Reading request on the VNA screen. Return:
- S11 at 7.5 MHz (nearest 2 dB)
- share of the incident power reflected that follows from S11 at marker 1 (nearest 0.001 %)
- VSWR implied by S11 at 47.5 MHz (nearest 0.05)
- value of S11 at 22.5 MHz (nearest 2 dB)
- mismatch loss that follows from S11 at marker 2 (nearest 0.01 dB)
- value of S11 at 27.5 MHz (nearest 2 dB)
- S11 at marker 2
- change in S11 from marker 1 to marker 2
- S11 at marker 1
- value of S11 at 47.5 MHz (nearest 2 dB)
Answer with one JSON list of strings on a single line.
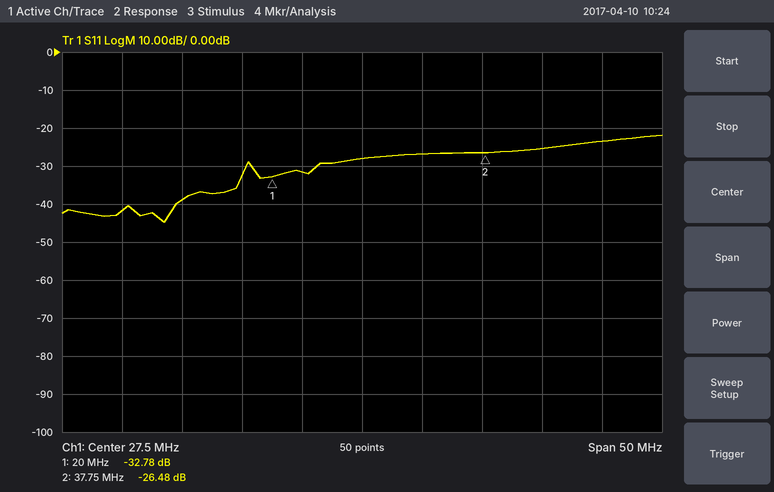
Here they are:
["-42 dB", "0.053 %", "1.15", "-32 dB", "0.01 dB", "-28 dB", "-26.48 dB", "6.30 dB", "-32.78 dB", "-24 dB"]
